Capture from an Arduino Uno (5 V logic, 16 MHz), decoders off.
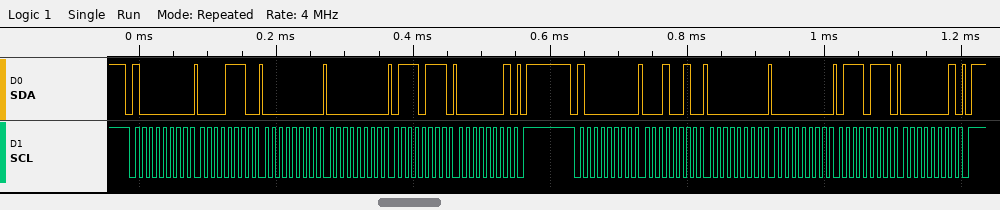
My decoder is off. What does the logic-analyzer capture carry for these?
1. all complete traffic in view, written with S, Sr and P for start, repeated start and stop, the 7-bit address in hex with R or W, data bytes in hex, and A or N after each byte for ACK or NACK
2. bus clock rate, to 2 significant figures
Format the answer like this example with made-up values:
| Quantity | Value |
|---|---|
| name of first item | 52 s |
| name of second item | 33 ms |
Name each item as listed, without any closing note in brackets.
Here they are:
| Quantity | Value |
|---|---|
| all complete traffic in view, written with S, Sr and P for start, repeated start and stop, the 7-bit address in hex with R or W, data bytes in hex, and A or N after each byte for ACK or NACK | S 40W A 0E A 00 A 00 A 77 A 01 A P S 40W A 12 A 00 A 00 A 77 A 01 A P |
| bus clock rate, to 2 significant figures | 100 kHz |
